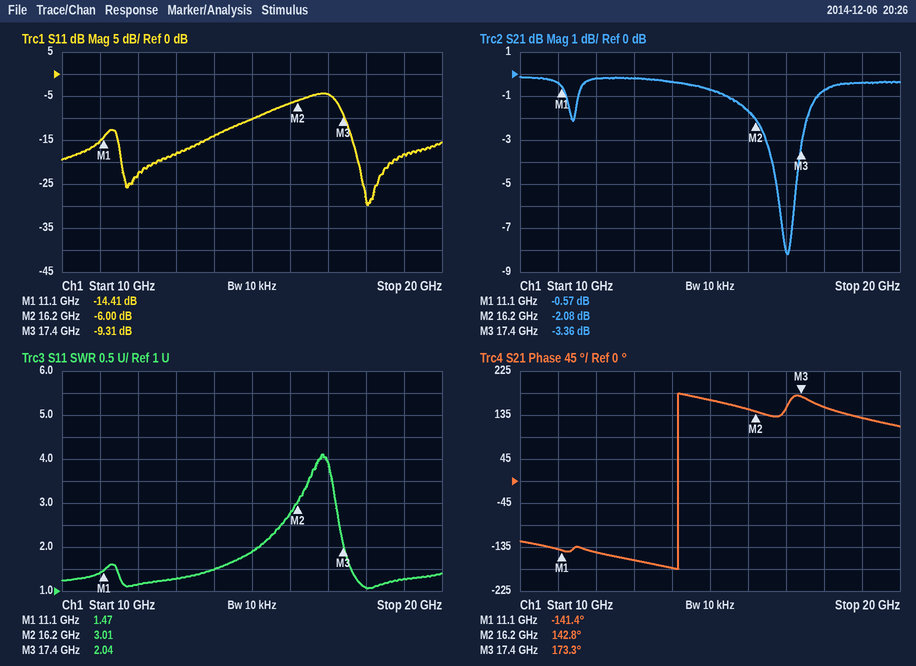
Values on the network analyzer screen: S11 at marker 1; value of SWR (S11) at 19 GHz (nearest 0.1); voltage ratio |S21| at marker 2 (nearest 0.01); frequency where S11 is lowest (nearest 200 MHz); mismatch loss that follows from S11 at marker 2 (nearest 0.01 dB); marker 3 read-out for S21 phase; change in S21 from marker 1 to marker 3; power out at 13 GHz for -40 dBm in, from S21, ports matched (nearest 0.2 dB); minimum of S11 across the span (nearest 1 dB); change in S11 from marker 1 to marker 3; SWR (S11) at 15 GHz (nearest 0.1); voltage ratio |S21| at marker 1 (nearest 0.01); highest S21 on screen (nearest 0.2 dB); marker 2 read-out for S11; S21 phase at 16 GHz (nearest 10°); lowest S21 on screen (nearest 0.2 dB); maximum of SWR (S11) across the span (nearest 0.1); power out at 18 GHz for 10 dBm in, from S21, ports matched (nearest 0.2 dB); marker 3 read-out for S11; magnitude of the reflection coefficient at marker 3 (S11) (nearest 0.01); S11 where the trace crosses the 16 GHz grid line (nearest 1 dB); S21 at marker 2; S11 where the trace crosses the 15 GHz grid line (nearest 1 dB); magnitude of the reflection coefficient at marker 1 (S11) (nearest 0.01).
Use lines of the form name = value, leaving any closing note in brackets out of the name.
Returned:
S11 at marker 1 = -14.41 dB
value of SWR (S11) at 19 GHz = 1.3
voltage ratio |S21| at marker 2 = 0.79
frequency where S11 is lowest = 18.0 GHz
mismatch loss that follows from S11 at marker 2 = 1.26 dB
marker 3 read-out for S21 phase = 173.3°
change in S21 from marker 1 to marker 3 = -2.79 dB
power out at 13 GHz for -40 dBm in, from S21, ports matched = -40.2 dBm
minimum of S11 across the span = -30 dB
change in S11 from marker 1 to marker 3 = 5.10 dB
SWR (S11) at 15 GHz = 1.9
voltage ratio |S21| at marker 1 = 0.94
highest S21 on screen = -0.2 dB
marker 2 read-out for S11 = -6.00 dB
S21 phase at 16 GHz = 150°
lowest S21 on screen = -8.2 dB
maximum of SWR (S11) across the span = 4.1
power out at 18 GHz for 10 dBm in, from S21, ports matched = 9.2 dBm
marker 3 read-out for S11 = -9.31 dB
magnitude of the reflection coefficient at marker 3 (S11) = 0.34
S11 where the trace crosses the 16 GHz grid line = -7 dB
S21 at marker 2 = -2.08 dB
S11 where the trace crosses the 15 GHz grid line = -10 dB
magnitude of the reflection coefficient at marker 1 (S11) = 0.19
